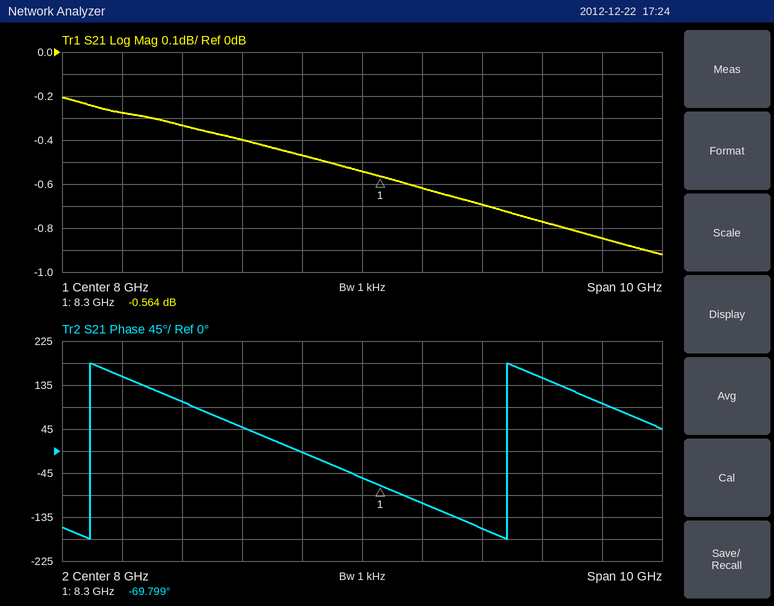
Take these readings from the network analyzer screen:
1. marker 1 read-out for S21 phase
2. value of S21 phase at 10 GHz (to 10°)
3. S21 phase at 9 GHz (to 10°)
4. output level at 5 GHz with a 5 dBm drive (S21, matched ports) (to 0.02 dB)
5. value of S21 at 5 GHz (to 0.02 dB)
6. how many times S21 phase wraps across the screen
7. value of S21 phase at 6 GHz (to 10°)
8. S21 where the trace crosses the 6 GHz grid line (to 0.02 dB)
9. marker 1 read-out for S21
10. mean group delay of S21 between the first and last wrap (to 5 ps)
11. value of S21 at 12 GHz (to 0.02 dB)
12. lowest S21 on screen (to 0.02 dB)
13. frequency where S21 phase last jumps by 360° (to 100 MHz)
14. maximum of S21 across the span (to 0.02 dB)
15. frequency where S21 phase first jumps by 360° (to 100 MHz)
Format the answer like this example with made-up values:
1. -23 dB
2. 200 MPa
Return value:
1. -69.799°
2. -160°
3. -110°
4. 4.66 dBm
5. -0.34 dB
6. 2
7. 50°
8. -0.40 dB
9. -0.564 dB
10. 145 ps
11. -0.84 dB
12. -0.92 dB
13. 10.4 GHz
14. -0.20 dB
15. 3.5 GHz
